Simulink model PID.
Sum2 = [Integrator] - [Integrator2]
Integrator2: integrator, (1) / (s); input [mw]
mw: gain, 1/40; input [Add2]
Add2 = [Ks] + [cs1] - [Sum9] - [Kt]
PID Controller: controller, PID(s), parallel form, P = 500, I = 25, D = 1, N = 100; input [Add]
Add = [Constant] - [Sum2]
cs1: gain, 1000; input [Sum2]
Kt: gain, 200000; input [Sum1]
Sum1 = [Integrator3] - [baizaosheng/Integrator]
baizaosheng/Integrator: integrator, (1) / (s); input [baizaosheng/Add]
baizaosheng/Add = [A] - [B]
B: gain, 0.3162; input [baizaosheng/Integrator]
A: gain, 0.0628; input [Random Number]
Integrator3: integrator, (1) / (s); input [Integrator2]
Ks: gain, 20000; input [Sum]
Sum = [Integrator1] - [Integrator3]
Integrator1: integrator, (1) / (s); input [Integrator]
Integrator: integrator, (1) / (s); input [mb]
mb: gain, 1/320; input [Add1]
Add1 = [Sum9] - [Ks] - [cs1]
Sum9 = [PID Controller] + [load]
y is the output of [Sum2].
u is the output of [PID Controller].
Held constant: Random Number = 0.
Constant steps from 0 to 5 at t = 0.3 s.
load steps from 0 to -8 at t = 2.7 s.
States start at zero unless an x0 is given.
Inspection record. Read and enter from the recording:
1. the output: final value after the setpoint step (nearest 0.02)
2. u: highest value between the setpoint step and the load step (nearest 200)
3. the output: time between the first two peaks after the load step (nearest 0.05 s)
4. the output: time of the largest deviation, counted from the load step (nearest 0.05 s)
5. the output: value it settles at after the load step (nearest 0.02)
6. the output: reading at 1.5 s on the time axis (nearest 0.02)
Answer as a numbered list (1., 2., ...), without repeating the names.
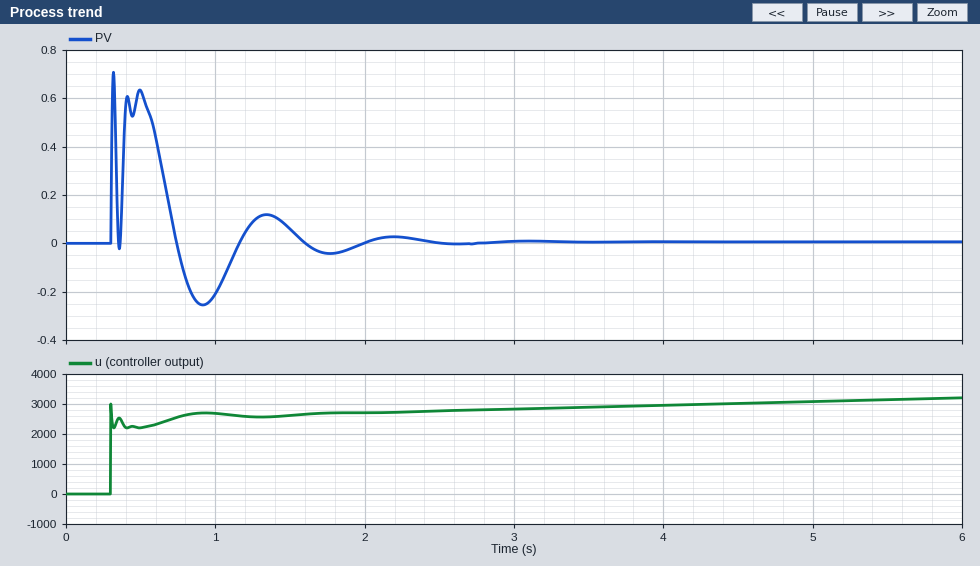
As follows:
1. 0.00
2. 3000
3. 0.85 s
4. 0.40 s
5. 0.00
6. 0.06
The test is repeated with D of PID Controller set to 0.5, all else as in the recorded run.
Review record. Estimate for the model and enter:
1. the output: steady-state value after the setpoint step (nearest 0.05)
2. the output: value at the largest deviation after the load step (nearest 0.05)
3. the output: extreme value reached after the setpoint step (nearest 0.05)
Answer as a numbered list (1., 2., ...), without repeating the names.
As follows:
1. 0.00
2. 0.00
3. 0.70
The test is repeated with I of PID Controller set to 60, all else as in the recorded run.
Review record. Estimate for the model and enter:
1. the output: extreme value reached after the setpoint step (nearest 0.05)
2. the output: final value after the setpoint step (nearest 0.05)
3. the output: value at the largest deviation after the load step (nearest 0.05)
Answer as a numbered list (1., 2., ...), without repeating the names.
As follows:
1. 0.70
2. 0.00
3. 0.00
